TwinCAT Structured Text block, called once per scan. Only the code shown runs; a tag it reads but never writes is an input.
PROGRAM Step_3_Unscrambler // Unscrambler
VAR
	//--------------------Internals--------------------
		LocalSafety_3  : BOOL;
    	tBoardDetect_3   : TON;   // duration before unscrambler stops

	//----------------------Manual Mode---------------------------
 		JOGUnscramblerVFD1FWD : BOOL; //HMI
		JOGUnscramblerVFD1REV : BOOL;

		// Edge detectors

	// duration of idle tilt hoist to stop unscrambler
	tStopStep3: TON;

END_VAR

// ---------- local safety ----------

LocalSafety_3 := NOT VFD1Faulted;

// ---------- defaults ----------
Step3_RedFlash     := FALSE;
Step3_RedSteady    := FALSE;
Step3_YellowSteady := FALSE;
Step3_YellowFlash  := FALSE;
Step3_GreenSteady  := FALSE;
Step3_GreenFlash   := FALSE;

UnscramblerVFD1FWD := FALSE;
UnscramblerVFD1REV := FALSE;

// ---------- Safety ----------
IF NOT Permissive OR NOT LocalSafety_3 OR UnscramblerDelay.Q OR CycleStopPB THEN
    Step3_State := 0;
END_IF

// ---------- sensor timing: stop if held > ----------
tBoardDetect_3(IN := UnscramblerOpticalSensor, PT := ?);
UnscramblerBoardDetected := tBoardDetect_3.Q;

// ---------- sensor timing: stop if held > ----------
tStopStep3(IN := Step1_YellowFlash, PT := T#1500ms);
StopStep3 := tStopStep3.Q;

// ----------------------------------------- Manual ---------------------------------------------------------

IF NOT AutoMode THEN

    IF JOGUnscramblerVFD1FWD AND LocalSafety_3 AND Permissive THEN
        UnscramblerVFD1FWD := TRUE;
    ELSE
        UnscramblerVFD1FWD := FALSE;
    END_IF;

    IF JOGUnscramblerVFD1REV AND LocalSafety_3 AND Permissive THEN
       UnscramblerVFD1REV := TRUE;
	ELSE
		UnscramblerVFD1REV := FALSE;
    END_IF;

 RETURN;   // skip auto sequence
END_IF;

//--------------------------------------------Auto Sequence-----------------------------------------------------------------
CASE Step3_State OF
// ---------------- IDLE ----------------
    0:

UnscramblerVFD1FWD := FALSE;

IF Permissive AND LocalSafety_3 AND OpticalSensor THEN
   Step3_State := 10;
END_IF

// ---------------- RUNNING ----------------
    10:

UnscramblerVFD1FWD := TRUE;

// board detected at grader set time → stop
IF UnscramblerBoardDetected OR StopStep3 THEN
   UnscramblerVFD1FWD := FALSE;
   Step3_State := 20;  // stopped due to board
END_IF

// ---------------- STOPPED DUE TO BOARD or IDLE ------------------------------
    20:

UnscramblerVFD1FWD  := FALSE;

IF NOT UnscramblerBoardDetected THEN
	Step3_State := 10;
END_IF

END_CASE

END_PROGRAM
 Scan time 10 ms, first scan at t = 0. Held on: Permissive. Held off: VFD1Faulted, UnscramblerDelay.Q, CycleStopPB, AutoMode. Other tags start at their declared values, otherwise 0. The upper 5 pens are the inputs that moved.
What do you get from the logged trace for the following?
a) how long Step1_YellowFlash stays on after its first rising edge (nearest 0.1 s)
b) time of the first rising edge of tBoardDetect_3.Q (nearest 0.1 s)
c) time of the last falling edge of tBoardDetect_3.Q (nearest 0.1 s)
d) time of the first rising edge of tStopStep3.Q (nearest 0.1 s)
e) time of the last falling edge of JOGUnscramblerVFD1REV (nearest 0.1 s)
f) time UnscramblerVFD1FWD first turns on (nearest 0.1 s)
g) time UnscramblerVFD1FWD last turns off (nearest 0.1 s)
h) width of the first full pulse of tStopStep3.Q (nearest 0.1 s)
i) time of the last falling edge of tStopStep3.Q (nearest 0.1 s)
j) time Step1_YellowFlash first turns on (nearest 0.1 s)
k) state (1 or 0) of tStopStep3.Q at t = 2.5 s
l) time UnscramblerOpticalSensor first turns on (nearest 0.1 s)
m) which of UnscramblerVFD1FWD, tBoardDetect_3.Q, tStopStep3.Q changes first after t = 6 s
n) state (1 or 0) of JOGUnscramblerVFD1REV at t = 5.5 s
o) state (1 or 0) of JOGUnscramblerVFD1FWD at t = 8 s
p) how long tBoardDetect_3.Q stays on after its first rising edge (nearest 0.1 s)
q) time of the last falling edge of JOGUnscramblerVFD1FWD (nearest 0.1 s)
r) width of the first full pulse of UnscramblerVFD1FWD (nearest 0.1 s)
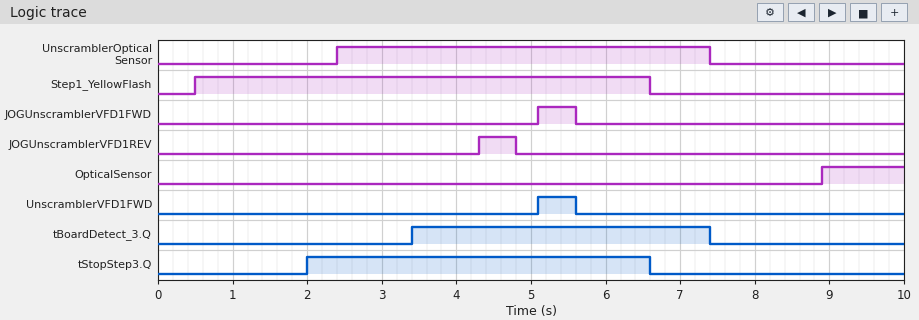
6.1 s
3.4 s
7.4 s
2.0 s
4.8 s
5.1 s
5.6 s
4.6 s
6.6 s
0.5 s
1
2.4 s
tStopStep3.Q
0
0
4.0 s
5.6 s
0.5 s
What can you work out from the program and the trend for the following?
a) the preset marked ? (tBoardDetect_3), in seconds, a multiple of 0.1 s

1.0 s
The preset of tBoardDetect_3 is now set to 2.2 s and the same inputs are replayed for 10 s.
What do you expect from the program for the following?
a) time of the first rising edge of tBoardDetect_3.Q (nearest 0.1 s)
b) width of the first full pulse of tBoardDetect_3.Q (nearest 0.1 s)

4.6 s
2.8 s
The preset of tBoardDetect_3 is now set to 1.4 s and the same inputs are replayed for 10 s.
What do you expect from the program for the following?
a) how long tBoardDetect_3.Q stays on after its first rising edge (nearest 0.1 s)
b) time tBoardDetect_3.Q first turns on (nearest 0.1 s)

3.6 s
3.8 s
